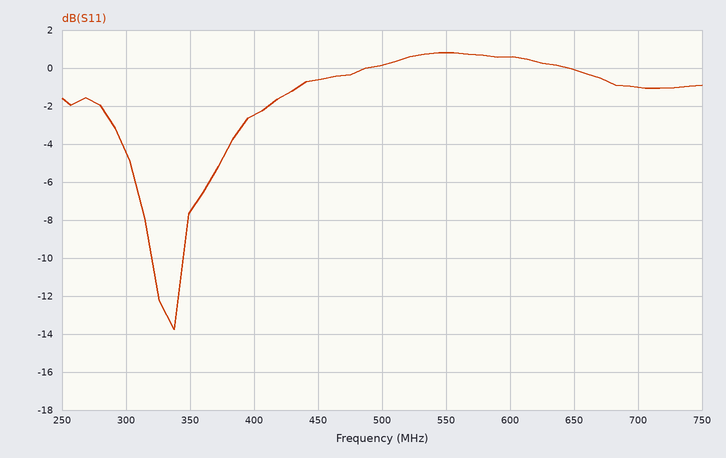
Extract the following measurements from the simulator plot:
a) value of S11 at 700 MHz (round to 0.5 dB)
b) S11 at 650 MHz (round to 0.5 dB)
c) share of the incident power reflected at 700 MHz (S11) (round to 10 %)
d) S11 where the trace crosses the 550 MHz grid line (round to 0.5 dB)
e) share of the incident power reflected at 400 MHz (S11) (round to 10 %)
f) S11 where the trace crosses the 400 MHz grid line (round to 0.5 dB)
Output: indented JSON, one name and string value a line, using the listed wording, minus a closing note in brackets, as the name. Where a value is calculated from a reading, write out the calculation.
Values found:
{
  "value of S11 at 700 MHz": "-1.0 dB",
  "S11 at 650 MHz": "0.0 dB",
  "share of the incident power reflected at 700 MHz (S11)": "10^(-1/10) ≈ 79.4 %, so 80 % to the nearest 10 %",
  "S11 where the trace crosses the 550 MHz grid line": "1.0 dB",
  "share of the incident power reflected at 400 MHz (S11)": "10^(-2.5/10) ≈ 56.2 %, so 60 % to the nearest 10 %",
  "S11 where the trace crosses the 400 MHz grid line": "-2.5 dB"
}
